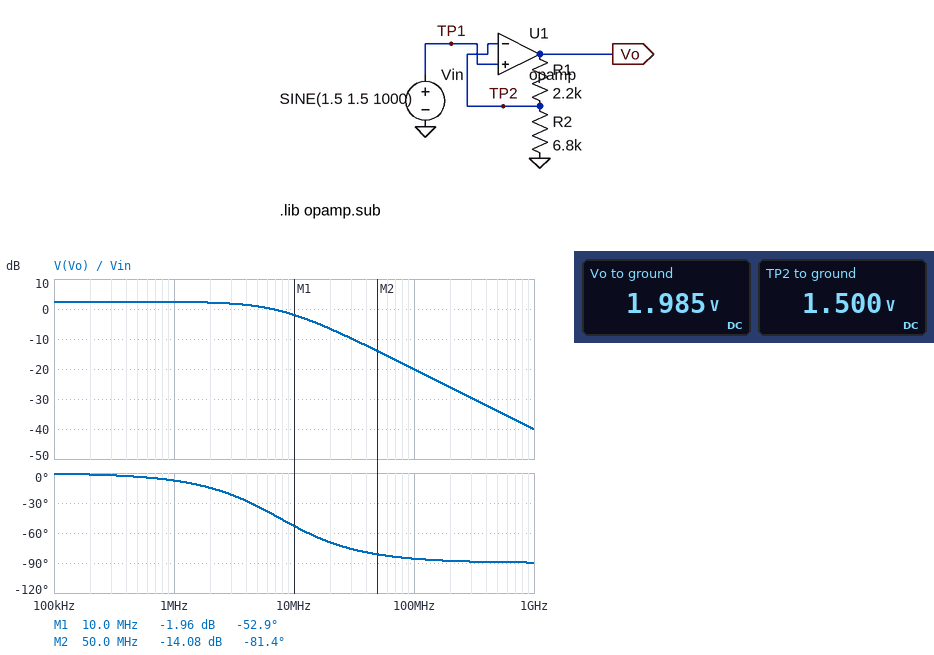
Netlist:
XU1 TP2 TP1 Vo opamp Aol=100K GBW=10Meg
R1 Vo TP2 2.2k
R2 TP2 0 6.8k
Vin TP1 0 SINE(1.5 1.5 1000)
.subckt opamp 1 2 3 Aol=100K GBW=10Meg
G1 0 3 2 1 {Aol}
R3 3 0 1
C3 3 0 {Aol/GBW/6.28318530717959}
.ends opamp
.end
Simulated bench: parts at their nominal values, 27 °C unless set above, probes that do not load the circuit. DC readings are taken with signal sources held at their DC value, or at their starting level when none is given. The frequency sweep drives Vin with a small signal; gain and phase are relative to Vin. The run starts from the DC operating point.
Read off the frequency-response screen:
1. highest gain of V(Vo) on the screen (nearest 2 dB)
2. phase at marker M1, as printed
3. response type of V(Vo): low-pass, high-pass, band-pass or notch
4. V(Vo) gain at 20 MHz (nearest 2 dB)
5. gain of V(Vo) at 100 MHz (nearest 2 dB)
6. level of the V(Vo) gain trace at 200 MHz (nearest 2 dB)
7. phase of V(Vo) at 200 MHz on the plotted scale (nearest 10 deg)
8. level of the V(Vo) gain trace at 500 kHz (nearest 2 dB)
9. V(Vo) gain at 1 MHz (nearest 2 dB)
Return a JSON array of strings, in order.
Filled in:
["2 dB", "-52.9 deg", "low-pass", "-6 dB", "-20 dB", "-26 dB", "-90 deg", "2 dB", "2 dB"]
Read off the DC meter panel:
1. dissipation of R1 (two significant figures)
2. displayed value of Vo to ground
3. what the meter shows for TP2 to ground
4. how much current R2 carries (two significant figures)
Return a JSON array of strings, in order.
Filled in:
["110 µW", "1.985 V", "1.500 V", "220 µA"]
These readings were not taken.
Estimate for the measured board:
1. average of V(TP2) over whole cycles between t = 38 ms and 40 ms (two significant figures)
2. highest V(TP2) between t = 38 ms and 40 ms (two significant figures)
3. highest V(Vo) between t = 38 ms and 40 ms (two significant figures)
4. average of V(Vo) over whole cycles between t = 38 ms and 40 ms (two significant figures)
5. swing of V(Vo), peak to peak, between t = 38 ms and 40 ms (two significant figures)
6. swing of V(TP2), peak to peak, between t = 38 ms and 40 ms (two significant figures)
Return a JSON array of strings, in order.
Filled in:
["1.5 V", "3.0 V", "4.0 V", "2.0 V", "4.0 V", "3.0 V"]
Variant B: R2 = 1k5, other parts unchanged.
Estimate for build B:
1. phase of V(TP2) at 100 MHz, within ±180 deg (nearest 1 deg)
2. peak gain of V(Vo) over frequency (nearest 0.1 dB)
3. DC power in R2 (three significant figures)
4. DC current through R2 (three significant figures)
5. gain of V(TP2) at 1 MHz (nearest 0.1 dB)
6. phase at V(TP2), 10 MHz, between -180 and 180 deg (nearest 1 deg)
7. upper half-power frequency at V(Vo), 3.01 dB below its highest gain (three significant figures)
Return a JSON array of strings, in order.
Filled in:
["-88 deg", "7.8 dB", "1.50 mW", "1.00 mA", "-0.3 dB", "-68 deg", "4.05 MHz"]
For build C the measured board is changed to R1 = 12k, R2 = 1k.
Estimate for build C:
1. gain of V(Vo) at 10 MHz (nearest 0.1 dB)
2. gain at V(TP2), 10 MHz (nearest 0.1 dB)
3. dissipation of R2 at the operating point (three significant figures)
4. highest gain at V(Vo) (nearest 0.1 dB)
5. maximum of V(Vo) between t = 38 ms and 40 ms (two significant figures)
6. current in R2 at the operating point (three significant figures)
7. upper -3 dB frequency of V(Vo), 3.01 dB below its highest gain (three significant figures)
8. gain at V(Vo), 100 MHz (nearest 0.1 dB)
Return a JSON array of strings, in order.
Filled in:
["0 dB", "-22.3 dB", "2.25 mW", "22.3 dB", "39 V", "1.50 mA", "769 kHz", "-20.0 dB"]
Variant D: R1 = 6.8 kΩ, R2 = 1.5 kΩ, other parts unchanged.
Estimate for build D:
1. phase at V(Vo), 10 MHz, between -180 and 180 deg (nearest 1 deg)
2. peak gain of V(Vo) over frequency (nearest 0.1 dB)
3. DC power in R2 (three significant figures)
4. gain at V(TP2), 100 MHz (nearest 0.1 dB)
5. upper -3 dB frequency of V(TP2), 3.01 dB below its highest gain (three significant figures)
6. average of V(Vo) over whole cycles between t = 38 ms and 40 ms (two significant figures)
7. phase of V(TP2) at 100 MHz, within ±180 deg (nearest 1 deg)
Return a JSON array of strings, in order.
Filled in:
["-80 deg", "14.9 dB", "1.50 mW", "-34.9 dB", "1.81 MHz", "8.3 V", "-89 deg"]
